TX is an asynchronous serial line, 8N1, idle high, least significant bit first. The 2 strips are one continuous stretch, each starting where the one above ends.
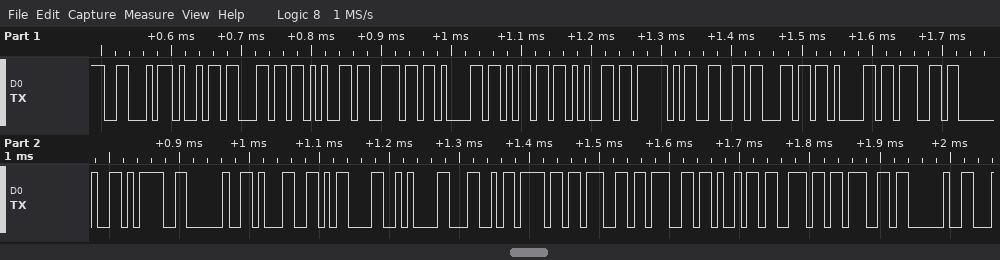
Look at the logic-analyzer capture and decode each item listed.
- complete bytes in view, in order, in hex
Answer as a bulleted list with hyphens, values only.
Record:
- 46 69 6C 65 6E 61 6D 65 5F 66 6C 61 67 20 3D 20 31 0D 0A 4C 6F 67 67 69 6E 67 20
